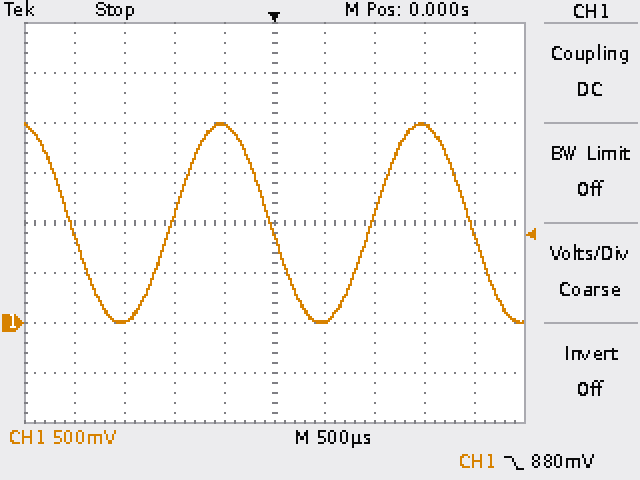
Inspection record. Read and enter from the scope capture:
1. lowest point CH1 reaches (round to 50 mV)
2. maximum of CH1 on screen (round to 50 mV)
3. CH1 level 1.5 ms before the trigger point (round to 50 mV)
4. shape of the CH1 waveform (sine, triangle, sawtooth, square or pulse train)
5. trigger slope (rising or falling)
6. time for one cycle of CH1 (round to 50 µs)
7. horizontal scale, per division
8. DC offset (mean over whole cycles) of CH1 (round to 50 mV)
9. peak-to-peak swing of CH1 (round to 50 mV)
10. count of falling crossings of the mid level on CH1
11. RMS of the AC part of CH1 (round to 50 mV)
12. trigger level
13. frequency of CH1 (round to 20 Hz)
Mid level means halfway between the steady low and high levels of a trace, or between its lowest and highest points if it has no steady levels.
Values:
0 mV
2.00 V
0 mV
sine
falling
2.00 ms
500 µs
1.00 V
2.00 V
3
700 mV
880 mV
500 Hz
